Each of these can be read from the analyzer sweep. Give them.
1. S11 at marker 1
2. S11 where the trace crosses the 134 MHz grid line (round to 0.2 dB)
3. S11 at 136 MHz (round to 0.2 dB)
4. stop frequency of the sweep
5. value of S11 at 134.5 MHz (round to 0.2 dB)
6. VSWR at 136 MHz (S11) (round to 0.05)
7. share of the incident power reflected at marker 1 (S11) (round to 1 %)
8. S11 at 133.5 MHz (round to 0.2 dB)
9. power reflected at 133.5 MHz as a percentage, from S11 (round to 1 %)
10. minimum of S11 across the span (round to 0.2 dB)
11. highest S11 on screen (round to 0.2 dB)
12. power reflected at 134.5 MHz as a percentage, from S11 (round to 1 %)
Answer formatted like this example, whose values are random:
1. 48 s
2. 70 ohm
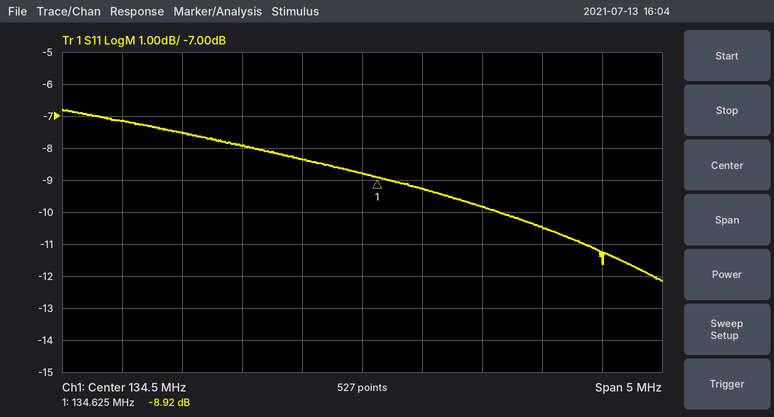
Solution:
1. -8.92 dB
2. -8.4 dB
3. -10.4 dB
4. 137 MHz
5. -8.8 dB
6. 1.85
7. 13 %
8. -8.0 dB
9. 16 %
10. -12.2 dB
11. -6.8 dB
12. 13 %
